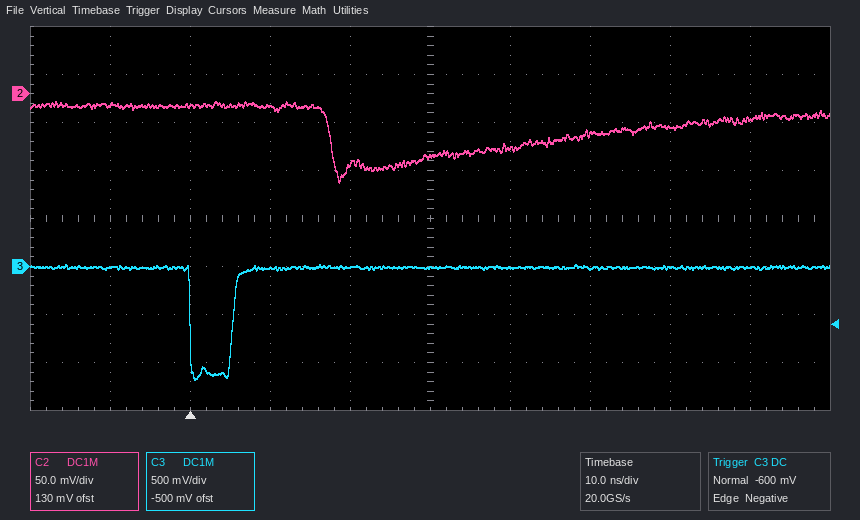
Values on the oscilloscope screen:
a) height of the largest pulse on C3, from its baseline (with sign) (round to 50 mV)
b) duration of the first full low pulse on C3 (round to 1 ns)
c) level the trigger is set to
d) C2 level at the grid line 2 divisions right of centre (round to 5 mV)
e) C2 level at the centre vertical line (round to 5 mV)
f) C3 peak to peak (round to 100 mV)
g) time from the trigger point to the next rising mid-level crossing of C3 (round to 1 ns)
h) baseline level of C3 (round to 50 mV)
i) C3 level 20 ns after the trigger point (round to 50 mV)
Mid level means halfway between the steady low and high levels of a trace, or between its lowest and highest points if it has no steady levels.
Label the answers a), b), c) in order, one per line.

a) -1.15 V
b) 5 ns
c) -600 mV
d) -40 mV
e) -65 mV
f) 1.20 V
g) 5 ns
h) 0 mV
i) 0 mV
